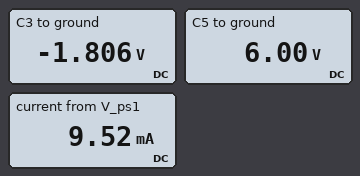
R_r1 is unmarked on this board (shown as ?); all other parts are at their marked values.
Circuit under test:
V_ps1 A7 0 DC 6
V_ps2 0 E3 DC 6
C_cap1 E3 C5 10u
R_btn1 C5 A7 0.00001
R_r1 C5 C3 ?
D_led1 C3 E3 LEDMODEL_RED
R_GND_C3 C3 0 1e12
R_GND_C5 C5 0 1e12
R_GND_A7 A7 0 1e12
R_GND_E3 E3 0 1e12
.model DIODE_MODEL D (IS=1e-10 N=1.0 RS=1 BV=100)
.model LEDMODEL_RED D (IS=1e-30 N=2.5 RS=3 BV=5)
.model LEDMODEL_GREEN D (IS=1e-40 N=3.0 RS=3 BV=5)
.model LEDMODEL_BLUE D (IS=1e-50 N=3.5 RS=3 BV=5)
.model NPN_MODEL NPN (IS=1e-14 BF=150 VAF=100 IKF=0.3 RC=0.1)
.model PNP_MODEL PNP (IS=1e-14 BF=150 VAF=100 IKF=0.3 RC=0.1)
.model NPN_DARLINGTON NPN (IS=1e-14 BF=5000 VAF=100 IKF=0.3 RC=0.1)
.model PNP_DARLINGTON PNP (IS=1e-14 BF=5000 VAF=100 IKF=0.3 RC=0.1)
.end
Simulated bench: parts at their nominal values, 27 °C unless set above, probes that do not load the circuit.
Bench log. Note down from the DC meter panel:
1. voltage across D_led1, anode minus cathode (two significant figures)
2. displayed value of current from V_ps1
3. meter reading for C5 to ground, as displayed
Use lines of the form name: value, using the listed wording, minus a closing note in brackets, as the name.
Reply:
voltage across D_led1, anode minus cathode: 4.2 V
displayed value of current from V_ps1: 9.52 mA
meter reading for C5 to ground, as displayed: 6.00 V
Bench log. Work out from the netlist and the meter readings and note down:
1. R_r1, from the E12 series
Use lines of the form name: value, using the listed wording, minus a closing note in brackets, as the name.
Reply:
R_r1, from the E12 series: 820 Ω
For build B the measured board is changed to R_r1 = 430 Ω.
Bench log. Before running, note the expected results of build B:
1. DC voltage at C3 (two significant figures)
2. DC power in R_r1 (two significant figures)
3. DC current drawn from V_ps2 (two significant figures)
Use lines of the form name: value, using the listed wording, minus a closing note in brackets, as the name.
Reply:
DC voltage at C3: -1.7 V
DC power in R_r1: 140 mW
DC current drawn from V_ps2: 18 mA
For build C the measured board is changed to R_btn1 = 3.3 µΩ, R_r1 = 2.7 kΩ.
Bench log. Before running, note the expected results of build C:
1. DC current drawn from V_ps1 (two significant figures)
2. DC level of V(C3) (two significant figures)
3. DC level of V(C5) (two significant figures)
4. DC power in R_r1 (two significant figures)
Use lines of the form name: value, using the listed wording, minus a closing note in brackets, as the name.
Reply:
DC current drawn from V_ps1: 2.9 mA
DC level of V(C3): -1.9 V
DC level of V(C5): 6.0 V
DC power in R_r1: 23 mW
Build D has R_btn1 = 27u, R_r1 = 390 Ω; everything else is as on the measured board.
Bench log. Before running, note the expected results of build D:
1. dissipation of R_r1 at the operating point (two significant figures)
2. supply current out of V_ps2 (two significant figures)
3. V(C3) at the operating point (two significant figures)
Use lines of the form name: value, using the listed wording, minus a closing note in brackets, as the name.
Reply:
dissipation of R_r1 at the operating point: 150 mW
supply current out of V_ps2: 20 mA
V(C3) at the operating point: -1.7 V
